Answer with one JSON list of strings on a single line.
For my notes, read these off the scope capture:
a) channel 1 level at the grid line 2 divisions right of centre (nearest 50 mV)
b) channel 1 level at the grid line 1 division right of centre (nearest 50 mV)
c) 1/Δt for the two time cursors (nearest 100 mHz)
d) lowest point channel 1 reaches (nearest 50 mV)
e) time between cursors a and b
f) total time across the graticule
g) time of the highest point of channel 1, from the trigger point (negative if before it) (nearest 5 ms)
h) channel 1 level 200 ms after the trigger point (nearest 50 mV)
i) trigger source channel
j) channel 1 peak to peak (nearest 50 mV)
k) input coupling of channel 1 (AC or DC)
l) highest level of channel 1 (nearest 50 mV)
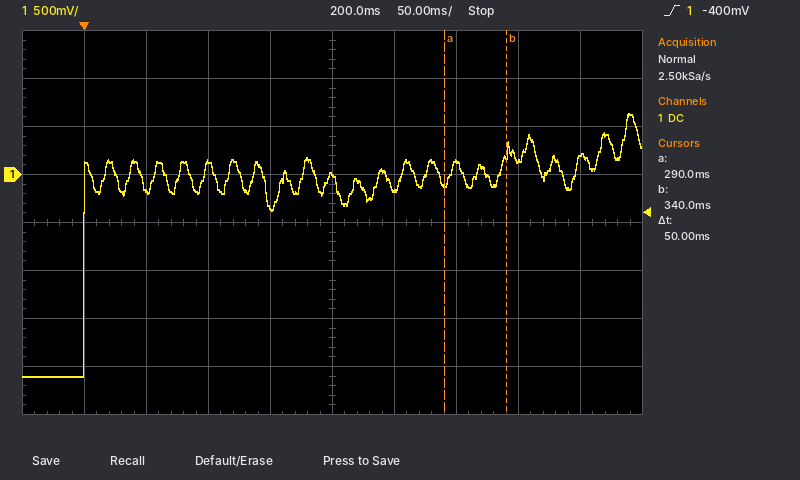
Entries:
["150 mV", "-150 mV", "20.0 Hz", "-2.10 V", "50 ms", "500 ms", "+440 ms", "0 mV", "channel 1", "2.75 V", "DC", "650 mV"]
